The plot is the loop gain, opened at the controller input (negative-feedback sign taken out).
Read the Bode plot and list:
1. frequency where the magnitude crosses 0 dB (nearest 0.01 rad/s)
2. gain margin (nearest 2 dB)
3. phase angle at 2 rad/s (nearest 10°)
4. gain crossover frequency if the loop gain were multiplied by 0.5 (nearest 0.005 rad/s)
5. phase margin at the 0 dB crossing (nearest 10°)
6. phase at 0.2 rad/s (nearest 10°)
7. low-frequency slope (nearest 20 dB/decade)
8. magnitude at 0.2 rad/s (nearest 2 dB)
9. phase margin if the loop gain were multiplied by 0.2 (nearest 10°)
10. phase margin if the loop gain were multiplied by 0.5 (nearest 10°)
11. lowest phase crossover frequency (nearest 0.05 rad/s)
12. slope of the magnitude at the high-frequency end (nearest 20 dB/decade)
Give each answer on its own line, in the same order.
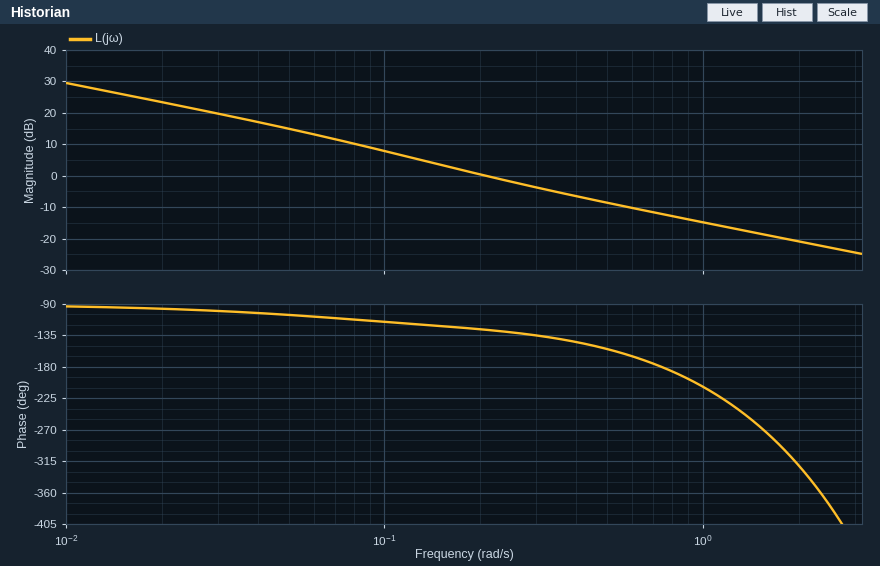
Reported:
0.21 rad/s
12 dB
-320°
0.120 rad/s
50°
-130°
-20 dB/decade
0 dB
70°
60°
0.75 rad/s
-20 dB/decade
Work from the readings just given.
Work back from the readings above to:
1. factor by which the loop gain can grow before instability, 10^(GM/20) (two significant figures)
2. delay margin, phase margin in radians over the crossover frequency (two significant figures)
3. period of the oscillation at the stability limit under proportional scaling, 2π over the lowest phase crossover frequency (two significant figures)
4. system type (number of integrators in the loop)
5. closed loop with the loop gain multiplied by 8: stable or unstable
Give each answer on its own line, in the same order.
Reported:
4.0
4.2 s
8.4 s
1
unstable
